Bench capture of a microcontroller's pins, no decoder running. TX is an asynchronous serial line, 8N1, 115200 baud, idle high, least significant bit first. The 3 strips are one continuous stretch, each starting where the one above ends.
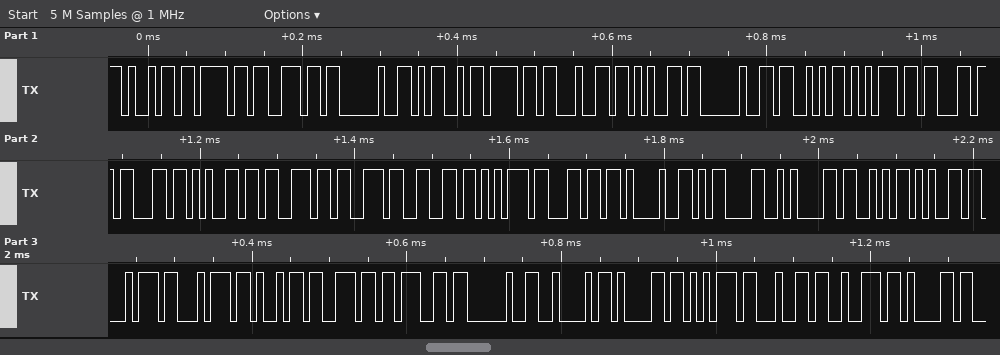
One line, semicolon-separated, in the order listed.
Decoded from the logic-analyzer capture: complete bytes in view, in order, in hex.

69 6F 6E 20 4D 6F 64 65 20 53 75 63 63 65 73 73 66 75 6C 21 0D 0A 53 65 74 74 69 6E 67 20 42 61 75 64 72 61
